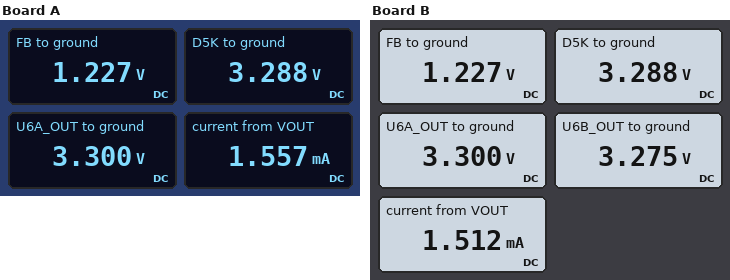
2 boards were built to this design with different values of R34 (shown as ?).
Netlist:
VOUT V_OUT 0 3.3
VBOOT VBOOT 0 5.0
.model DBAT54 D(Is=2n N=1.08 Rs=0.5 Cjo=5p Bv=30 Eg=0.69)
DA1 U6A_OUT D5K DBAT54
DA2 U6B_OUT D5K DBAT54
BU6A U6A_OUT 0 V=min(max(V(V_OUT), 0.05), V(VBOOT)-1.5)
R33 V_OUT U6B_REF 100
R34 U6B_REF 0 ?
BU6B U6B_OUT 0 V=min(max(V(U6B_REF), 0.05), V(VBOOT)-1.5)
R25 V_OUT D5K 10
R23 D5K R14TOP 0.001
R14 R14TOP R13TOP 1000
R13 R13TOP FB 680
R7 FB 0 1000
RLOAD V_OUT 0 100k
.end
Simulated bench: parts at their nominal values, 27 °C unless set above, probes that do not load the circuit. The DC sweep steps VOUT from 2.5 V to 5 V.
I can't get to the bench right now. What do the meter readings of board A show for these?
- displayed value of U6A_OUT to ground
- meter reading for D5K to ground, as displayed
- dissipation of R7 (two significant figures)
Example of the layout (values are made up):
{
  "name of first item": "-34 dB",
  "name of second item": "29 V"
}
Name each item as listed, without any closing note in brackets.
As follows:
{
  "displayed value of U6A_OUT to ground": "3.300 V",
  "meter reading for D5K to ground, as displayed": "3.288 V",
  "dissipation of R7": "1.5 mW"
}
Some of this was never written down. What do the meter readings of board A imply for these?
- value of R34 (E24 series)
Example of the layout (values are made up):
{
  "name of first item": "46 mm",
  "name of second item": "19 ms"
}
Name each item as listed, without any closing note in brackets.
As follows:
{
  "value of R34": "11 kΩ"
}
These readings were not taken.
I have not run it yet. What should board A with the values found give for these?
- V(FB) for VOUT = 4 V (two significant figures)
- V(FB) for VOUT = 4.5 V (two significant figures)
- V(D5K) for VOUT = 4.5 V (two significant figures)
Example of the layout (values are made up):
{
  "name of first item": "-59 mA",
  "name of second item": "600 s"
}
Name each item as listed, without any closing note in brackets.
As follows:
{
  "V(FB) for VOUT = 4 V": "1.5 V",
  "V(FB) for VOUT = 4.5 V": "1.7 V",
  "V(D5K) for VOUT = 4.5 V": "4.5 V"
}
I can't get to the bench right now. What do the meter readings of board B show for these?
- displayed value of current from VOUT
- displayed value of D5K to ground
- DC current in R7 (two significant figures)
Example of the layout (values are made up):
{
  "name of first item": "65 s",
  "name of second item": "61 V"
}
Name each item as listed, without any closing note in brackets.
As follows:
{
  "displayed value of current from VOUT": "1.512 mA",
  "displayed value of D5K to ground": "3.288 V",
  "DC current in R7": "1.2 mA"
}
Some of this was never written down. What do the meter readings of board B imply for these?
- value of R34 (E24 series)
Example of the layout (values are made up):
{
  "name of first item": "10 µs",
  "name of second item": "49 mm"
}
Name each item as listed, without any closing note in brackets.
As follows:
{
  "value of R34": "13 kΩ"
}
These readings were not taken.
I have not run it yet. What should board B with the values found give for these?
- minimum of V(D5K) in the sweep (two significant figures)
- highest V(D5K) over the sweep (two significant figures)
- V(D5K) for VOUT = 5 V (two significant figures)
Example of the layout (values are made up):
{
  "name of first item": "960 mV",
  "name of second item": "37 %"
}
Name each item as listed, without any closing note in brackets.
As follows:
{
  "minimum of V(D5K) in the sweep": "2.5 V",
  "highest V(D5K) over the sweep": "5.0 V",
  "V(D5K) for VOUT = 5 V": "5.0 V"
}
